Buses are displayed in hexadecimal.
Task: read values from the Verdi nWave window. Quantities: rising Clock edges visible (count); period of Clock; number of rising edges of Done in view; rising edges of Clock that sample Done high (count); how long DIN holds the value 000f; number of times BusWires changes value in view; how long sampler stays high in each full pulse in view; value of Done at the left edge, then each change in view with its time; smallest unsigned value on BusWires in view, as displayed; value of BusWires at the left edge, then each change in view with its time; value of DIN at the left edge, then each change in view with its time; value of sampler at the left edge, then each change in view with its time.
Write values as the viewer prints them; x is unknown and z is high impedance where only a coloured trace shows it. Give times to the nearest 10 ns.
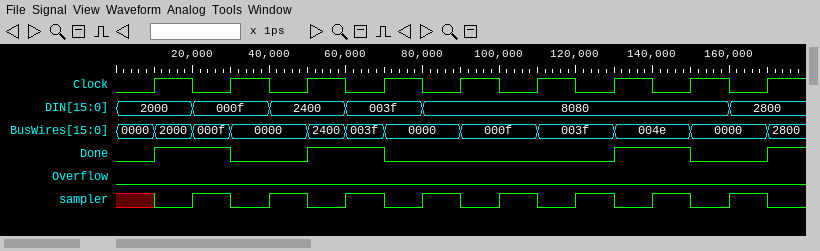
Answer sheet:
9
20 ns
4
3
20 ns
11
10 ns, 10 ns, 10 ns, 10 ns, 10 ns, 10 ns, 10 ns, 10 ns
0, 1 at 10 ns, 0 at 30 ns, 1 at 50 ns, 0 at 70 ns, 1 at 130 ns, 0 at 150 ns, 1 at 170 ns
0000
0000, 2000 at 10 ns, 000f at 20 ns, 0000 at 30 ns, 2400 at 50 ns, 003f at 60 ns, 0000 at 70 ns, 000f at 90 ns, 003f at 110 ns, 004e at 130 ns, 0000 at 150 ns, 2800 at 170 ns
2000, 000f at 20 ns, 2400 at 40 ns, 003f at 60 ns, 8080 at 80 ns, 2800 at 160 ns
x, 0 at 10 ns, 1 at 20 ns, 0 at 30 ns, 1 at 40 ns, 0 at 50 ns, 1 at 60 ns, 0 at 70 ns, 1 at 80 ns, 0 at 90 ns, 1 at 100 ns, 0 at 110 ns, 1 at 120 ns, 0 at 130 ns, 1 at 140 ns, 0 at 150 ns, 1 at 160 ns, 0 at 170 ns
